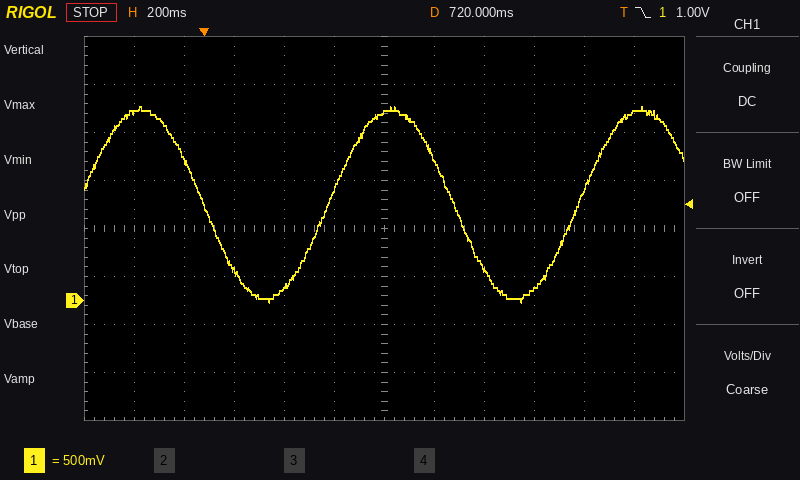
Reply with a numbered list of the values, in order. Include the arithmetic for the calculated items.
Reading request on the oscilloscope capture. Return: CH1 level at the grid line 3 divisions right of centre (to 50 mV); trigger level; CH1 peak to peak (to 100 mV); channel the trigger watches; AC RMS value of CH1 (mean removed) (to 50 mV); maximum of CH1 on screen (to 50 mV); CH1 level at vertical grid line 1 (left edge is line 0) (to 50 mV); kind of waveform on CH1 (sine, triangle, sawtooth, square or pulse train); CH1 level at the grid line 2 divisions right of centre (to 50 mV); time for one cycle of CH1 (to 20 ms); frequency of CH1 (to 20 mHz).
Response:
1. 100 mV
2. 1.00 V
3. 2.00 V
4. CH1
5. 2.00 V / (2√2) ≈ 707 mV, so 700 mV to the nearest 50 mV
6. 2.00 V
7. 1.95 V
8. sine
9. 350 mV
10. 1.00 s
11. 1 / 1.00 s ≈ 1.00 Hz
